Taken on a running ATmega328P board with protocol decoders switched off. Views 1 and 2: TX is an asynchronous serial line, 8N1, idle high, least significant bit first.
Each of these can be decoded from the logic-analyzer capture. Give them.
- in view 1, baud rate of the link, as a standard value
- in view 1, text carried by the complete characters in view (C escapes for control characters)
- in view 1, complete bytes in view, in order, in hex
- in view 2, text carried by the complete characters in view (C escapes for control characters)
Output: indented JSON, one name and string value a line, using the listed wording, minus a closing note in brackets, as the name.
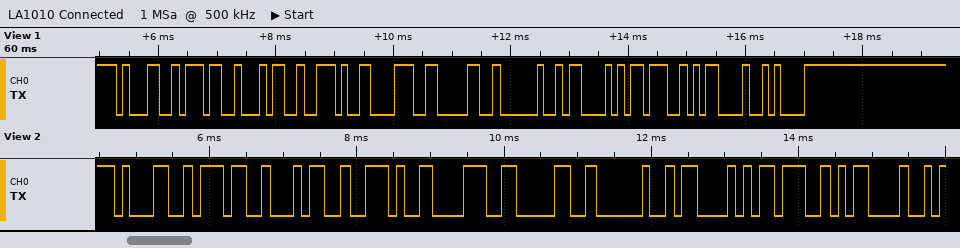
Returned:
{
  "in view 1, baud rate of the link, as a standard value": "9600 baud",
  "in view 1, text carried by the complete characters in view": "\"174.80 C;\\r\\n\"",
  "in view 1, complete bytes in view, in order, in hex": "0x31 0x37 0x34 0x2E 0x38 0x30 0x20 0x43 0x3B 0x0D 0x0A",
  "in view 2, text carried by the complete characters in view": "\"174.80 C;\\r\""
}
